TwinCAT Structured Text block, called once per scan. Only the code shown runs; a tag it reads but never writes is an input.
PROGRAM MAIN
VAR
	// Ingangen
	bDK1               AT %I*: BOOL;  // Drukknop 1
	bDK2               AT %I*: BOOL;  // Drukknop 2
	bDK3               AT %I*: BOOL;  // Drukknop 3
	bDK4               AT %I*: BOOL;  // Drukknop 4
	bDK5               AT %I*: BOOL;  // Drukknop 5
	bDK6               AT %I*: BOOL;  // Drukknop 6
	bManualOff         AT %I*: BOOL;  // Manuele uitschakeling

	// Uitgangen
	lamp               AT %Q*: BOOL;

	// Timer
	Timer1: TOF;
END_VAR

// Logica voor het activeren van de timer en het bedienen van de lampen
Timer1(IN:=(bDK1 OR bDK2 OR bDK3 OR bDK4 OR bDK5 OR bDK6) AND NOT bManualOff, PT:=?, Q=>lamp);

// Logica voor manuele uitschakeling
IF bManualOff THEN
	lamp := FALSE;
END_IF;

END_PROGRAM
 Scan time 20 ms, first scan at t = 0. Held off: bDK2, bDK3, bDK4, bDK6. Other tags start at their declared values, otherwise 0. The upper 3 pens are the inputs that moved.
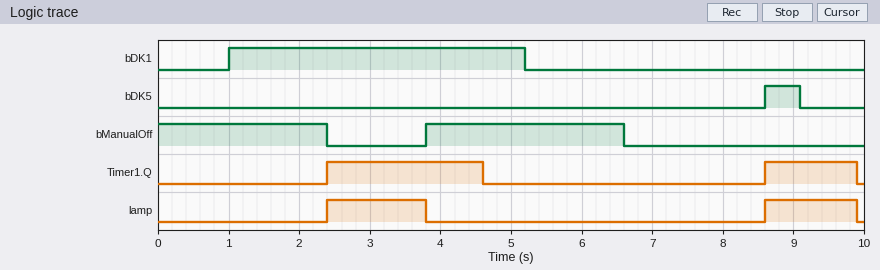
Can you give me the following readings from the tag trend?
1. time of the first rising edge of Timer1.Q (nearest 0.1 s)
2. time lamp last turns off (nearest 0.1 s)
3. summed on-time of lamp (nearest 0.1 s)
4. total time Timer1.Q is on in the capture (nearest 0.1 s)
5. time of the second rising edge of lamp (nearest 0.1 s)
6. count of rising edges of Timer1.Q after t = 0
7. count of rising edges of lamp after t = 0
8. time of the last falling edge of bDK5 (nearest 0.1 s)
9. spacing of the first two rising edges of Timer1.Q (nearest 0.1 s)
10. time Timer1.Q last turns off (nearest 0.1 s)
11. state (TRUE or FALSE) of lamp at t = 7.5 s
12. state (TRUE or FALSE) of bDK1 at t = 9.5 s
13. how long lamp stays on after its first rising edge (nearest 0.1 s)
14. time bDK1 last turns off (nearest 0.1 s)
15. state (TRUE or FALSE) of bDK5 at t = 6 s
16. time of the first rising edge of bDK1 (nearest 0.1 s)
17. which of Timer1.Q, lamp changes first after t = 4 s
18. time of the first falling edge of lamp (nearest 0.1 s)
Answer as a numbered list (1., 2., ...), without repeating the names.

1. 2.4 s
2. 9.9 s
3. 2.7 s
4. 3.5 s
5. 8.6 s
6. 2
7. 2
8. 9.1 s
9. 6.2 s
10. 9.9 s
11. FALSE
12. FALSE
13. 1.4 s
14. 5.2 s
15. FALSE
16. 1.0 s
17. Timer1.Q
18. 3.8 s
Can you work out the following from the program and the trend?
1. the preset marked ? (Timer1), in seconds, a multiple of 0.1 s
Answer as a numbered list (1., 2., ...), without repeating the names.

1. 0.8 s
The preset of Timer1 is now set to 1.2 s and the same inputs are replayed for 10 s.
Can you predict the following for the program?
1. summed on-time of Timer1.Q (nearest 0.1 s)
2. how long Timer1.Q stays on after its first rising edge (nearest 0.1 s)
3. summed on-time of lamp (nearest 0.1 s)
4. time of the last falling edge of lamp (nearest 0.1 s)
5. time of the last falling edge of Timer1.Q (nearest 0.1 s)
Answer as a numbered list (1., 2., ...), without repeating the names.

1. 4.0 s
2. 2.6 s
3. 2.8 s
4. 3.8 s
5. 5.0 s
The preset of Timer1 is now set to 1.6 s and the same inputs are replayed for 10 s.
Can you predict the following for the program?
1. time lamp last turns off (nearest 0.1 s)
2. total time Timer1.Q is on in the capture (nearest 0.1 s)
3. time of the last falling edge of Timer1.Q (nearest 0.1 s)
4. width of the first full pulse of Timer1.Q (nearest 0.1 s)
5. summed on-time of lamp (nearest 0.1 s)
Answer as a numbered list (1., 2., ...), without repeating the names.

1. 3.8 s
2. 4.4 s
3. 5.4 s
4. 3.0 s
5. 2.8 s
